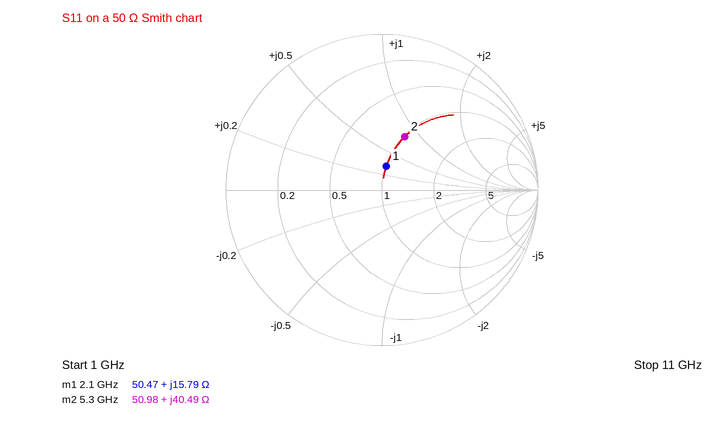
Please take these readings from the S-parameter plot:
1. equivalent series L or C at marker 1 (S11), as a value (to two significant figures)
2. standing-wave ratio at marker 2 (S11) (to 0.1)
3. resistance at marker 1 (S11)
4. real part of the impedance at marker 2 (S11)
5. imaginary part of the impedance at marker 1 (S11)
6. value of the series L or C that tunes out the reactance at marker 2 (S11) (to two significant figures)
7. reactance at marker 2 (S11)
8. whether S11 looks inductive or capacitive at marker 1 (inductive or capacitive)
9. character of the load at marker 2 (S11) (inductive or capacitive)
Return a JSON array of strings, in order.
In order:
["1.2 nH", "2.2", "50.47 Ω", "50.98 Ω", "+15.79 Ω", "740 fF", "+40.49 Ω", "inductive", "inductive"]
